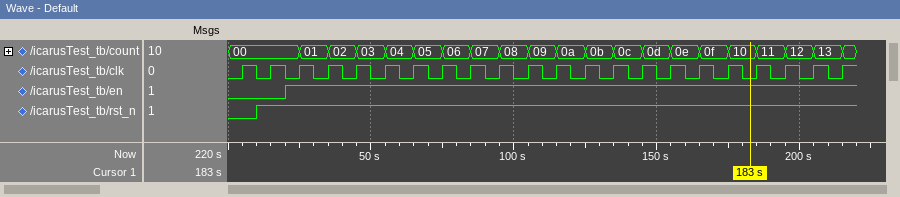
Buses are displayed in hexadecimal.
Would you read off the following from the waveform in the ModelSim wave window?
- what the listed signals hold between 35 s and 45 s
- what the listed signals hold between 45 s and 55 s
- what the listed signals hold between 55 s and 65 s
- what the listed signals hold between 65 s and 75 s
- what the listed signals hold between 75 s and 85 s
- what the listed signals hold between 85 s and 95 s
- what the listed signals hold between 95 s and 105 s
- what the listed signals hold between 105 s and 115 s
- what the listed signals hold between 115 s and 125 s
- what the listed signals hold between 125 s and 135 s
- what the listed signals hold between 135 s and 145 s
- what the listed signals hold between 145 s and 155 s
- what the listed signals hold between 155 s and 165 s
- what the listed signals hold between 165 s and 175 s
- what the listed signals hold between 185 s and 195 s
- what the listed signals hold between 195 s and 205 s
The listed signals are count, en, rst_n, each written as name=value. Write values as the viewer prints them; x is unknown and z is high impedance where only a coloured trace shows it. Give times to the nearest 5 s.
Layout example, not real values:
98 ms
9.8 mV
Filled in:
count=02, en=1, rst_n=1
count=03, en=1, rst_n=1
count=04, en=1, rst_n=1
count=05, en=1, rst_n=1
count=06, en=1, rst_n=1
count=07, en=1, rst_n=1
count=08, en=1, rst_n=1
count=09, en=1, rst_n=1
count=0a, en=1, rst_n=1
count=0b, en=1, rst_n=1
count=0c, en=1, rst_n=1
count=0d, en=1, rst_n=1
count=0e, en=1, rst_n=1
count=0f, en=1, rst_n=1
count=11, en=1, rst_n=1
count=12, en=1, rst_n=1
